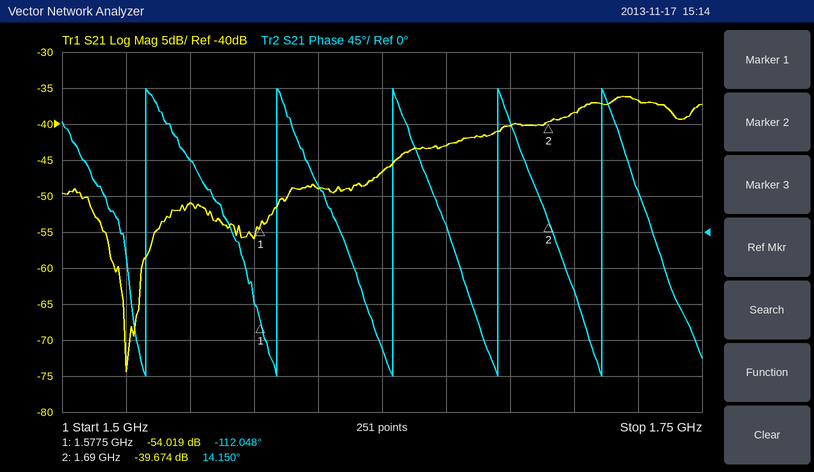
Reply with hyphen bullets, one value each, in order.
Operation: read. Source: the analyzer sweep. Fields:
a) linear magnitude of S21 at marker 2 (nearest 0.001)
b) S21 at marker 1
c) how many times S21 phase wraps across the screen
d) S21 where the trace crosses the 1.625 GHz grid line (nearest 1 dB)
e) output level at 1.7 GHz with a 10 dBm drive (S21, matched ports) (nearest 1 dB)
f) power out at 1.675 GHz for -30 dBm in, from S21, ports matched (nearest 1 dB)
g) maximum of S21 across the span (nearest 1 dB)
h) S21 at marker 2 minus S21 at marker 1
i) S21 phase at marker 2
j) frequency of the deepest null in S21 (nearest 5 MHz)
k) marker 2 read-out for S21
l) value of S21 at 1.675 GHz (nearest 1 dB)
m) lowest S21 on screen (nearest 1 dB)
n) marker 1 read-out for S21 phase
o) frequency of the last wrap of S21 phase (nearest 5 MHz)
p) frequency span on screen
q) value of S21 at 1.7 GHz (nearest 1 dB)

- 0.010
- -54.019 dB
- 5
- -47 dB
- -28 dBm
- -70 dBm
- -36 dB
- 14.345 dB
- 14.150°
- 1.525 GHz
- -39.674 dB
- -40 dB
- -74 dB
- -112.048°
- 1.710 GHz
- 250 MHz
- -38 dB
